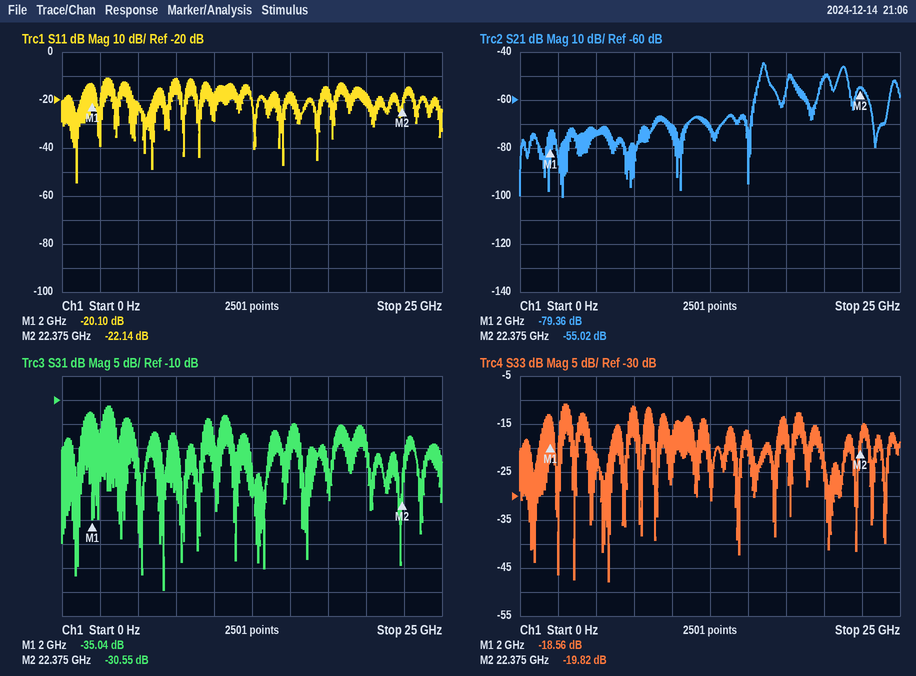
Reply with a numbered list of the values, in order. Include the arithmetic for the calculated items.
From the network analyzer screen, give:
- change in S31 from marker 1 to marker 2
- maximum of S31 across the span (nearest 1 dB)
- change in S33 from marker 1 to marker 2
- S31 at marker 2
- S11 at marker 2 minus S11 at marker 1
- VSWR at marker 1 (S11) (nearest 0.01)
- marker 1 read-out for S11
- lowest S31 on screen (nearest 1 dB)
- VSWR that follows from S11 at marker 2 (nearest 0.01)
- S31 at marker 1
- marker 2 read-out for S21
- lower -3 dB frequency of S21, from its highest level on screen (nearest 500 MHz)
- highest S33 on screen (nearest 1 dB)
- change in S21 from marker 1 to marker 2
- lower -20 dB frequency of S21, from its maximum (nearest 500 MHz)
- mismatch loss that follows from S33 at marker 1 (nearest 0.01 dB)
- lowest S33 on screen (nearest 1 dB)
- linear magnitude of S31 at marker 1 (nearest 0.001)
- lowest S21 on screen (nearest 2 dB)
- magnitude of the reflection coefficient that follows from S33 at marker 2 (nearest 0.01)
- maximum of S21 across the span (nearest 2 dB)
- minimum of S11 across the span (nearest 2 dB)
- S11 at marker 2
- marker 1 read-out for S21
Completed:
1. -30.55 − (-35.04) = 4.49 dB
2. -11 dB
3. -19.82 − (-18.56) = -1.26 dB
4. -30.55 dB
5. -22.14 − (-20.1) = -2.04 dB
6. (1 + 0.0989)/(1 − 0.0989) ≈ 1.22
7. -20.10 dB
8. -50 dB
9. (1 + 0.0782)/(1 − 0.0782) ≈ 1.17
10. -35.04 dB
11. -55.02 dB
12. 16.0 GHz
13. -11 dB
14. -55.02 − (-79.36) = 24.34 dB
15. 15.5 GHz
16. −10 log10(1 − 10^(-18.56/10)) ≈ 0.06 dB
17. -48 dB
18. 10^(-35.04/20) ≈ 0.018
19. -100 dB
20. 10^(-19.82/20) ≈ 0.10
21. -44 dB
22. -54 dB
23. -22.14 dB
24. -79.36 dB
